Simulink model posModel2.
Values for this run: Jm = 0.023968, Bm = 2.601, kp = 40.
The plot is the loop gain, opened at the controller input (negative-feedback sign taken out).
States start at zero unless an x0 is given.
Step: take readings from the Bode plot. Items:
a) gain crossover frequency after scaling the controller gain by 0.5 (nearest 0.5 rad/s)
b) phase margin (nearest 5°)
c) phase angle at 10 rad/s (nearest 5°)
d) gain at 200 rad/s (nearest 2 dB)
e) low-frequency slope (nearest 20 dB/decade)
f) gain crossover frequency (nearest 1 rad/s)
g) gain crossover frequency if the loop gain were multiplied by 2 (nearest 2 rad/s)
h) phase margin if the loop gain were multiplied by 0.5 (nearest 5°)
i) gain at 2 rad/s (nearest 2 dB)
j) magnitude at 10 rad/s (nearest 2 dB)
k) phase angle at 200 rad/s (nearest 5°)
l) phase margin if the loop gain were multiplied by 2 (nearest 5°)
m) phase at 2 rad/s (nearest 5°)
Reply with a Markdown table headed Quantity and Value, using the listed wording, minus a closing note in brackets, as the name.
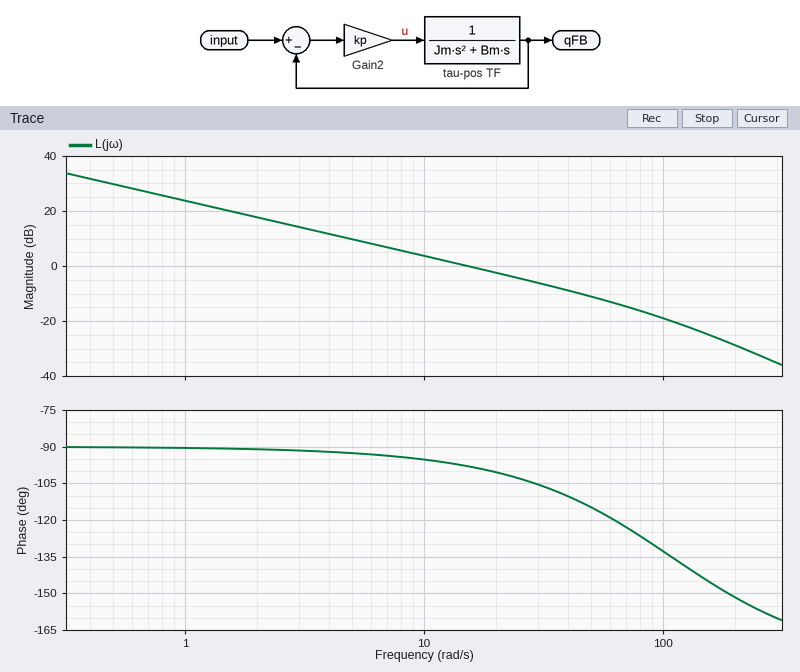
| Quantity | Value |
|---|---|
| gain crossover frequency after scaling the controller gain by 0.5 | 7.5 rad/s |
| phase margin | 80° |
| phase angle at 10 rad/s | -95° |
| gain at 200 rad/s | -28 dB |
| low-frequency slope | -20 dB/decade |
| gain crossover frequency | 15 rad/s |
| gain crossover frequency if the loop gain were multiplied by 2 | 30 rad/s |
| phase margin if the loop gain were multiplied by 0.5 | 85° |
| gain at 2 rad/s | 18 dB |
| magnitude at 10 rad/s | 4 dB |
| phase angle at 200 rad/s | -150° |
| phase margin if the loop gain were multiplied by 2 | 75° |
| phase at 2 rad/s | -90° |
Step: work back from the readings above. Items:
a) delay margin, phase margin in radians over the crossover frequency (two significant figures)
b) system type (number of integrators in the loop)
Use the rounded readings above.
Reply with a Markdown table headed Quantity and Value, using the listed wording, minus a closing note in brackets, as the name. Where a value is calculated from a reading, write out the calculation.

| Quantity | Value |
|---|---|
| delay margin, phase margin in radians over the crossover frequency | 80 × π / 180 / 15 = 0.093 s |
| system type | 1 |
